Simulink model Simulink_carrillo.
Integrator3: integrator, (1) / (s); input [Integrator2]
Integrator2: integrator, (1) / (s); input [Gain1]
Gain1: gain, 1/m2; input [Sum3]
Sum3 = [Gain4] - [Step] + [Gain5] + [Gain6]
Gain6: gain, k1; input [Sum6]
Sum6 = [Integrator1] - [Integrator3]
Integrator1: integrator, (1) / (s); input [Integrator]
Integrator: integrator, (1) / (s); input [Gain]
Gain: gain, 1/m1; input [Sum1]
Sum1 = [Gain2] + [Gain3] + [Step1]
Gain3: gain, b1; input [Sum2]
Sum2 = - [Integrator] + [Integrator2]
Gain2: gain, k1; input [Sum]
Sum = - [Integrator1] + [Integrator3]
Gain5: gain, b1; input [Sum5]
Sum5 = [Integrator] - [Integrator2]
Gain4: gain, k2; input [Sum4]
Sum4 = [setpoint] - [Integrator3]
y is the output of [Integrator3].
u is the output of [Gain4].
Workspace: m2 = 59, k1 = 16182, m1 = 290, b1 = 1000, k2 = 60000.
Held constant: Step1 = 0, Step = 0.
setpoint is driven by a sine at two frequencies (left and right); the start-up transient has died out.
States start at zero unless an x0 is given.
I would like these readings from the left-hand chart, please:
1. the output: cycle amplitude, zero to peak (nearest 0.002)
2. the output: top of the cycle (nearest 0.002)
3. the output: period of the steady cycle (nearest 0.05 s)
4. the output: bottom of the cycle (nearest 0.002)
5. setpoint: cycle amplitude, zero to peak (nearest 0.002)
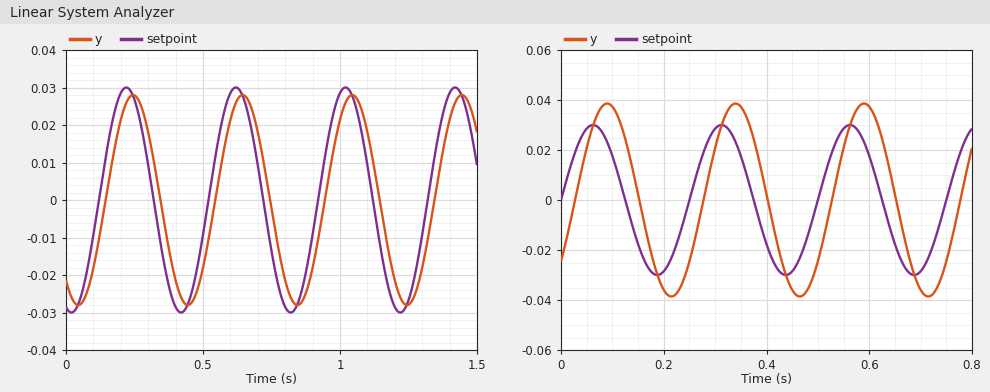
0.028
0.028
0.40 s
-0.028
0.030
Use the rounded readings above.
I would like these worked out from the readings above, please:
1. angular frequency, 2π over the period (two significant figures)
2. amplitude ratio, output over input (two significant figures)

16 rad/s
0.93
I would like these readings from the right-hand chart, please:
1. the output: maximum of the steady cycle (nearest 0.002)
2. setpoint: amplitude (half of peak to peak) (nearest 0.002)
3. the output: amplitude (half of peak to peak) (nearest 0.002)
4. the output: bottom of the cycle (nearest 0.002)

0.038
0.030
0.038
-0.038
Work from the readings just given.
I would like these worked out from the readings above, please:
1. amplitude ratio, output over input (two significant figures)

1.3
